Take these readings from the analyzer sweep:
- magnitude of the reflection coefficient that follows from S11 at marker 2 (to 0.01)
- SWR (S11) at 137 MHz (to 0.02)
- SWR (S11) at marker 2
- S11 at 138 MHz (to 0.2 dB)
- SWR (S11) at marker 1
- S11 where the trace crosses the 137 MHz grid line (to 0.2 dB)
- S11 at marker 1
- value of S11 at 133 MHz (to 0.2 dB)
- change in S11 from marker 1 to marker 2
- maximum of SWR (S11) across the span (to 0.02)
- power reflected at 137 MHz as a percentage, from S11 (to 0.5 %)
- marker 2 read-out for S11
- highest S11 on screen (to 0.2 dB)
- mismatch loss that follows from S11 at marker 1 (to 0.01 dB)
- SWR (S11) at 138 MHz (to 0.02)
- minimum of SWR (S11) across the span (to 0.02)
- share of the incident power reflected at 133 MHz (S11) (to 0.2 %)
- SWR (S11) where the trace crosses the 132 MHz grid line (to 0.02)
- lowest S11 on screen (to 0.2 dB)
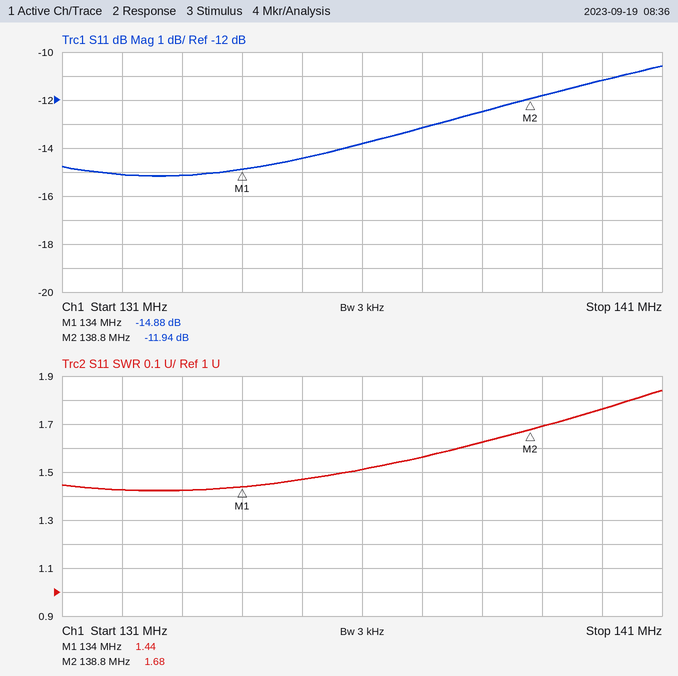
0.25
1.56
1.68
-12.4 dB
1.44
-13.2 dB
-14.88 dB
-15.2 dB
2.94 dB
1.84
5.0 %
-11.94 dB
-10.6 dB
0.14 dB
1.62
1.42
3.0 %
1.42
-15.2 dB
